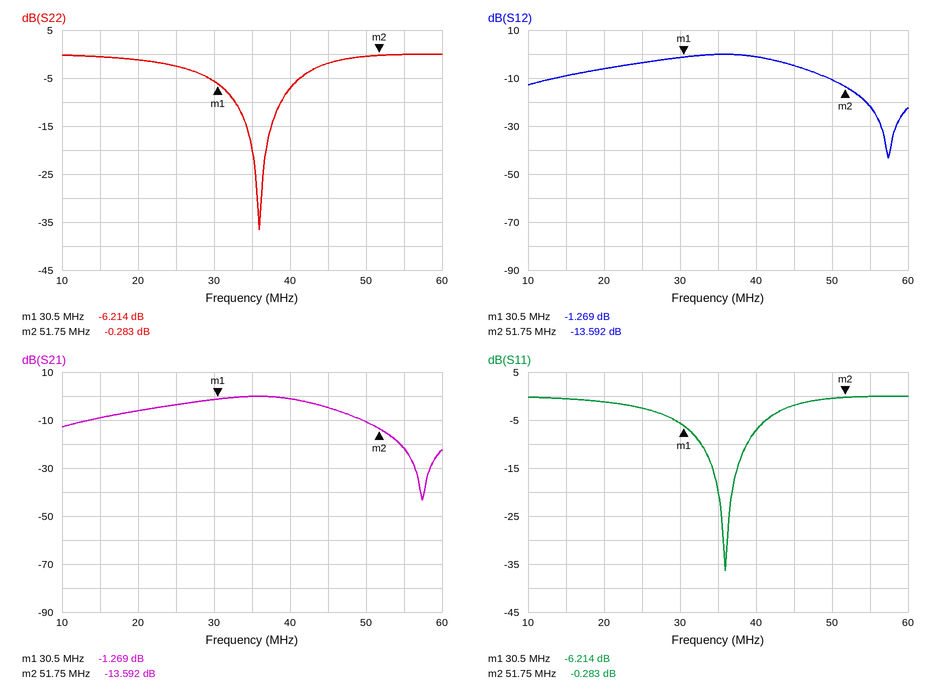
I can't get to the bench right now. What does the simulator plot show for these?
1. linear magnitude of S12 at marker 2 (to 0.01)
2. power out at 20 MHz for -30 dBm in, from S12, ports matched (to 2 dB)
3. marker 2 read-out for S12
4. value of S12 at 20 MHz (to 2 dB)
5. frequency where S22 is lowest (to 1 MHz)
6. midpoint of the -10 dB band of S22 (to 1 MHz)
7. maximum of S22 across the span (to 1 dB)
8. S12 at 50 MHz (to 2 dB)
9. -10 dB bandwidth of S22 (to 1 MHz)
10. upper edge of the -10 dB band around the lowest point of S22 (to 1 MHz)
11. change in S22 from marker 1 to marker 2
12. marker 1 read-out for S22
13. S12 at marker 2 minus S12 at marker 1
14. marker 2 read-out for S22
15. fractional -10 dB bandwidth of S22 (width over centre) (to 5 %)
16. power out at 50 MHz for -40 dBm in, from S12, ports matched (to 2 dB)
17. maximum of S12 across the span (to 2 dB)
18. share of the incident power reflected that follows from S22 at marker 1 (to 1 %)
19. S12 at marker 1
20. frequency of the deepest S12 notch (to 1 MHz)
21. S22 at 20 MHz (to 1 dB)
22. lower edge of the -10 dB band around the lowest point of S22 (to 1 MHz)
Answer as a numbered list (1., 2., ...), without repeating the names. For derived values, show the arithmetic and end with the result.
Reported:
1. 10^(-13.592/20) ≈ 0.21
2. -30 dBm + (-6 dB) = -36 dBm
3. -13.592 dB
4. -6 dB
5. 36 MHz
6. 36 MHz
7. 0 dB
8. -10 dB
9. 39 MHz − 33 MHz = 6 MHz
10. 39 MHz
11. -0.283 − (-6.214) = 5.931 dB
12. -6.214 dB
13. -13.592 − (-1.269) = -12.323 dB
14. -0.283 dB
15. 6 MHz / 36 MHz ≈ 16.7 %, so 15 % to the nearest 5 %
16. -40 dBm + (-10 dB) = -50 dBm
17. 0 dB
18. 10^(-6.214/10) ≈ 24 %
19. -1.269 dB
20. 57 MHz
21. -1 dB
22. 33 MHz
